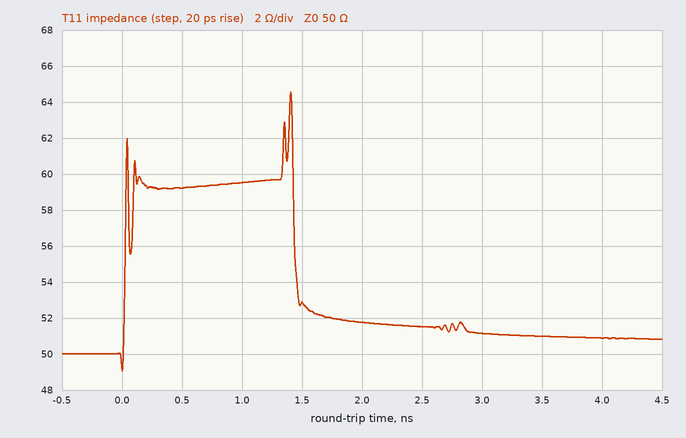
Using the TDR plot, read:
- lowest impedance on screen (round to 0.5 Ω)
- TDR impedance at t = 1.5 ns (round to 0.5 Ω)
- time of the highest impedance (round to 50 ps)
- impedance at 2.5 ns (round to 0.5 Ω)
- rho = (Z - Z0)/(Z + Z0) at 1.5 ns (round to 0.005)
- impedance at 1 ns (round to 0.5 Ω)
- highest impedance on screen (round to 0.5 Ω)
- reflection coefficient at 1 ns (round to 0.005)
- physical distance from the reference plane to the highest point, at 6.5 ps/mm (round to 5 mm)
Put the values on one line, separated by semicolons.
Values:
49.0 Ω; 53.0 Ω; 1.40 ns; 51.5 Ω; +0.030; 59.5 Ω; 64.5 Ω; +0.085; 110 mm
